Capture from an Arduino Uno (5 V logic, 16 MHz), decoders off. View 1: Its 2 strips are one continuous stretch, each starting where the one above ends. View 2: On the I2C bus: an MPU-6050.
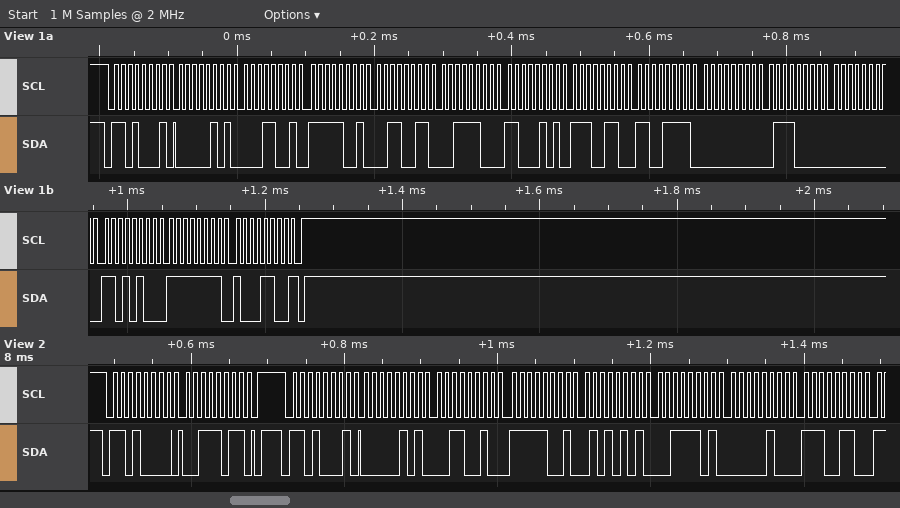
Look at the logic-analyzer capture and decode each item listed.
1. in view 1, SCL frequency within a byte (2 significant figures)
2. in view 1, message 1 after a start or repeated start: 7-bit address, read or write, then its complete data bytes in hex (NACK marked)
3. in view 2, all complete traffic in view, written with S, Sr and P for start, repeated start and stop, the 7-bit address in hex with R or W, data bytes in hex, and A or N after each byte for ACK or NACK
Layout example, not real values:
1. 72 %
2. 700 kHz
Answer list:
1. 100 kHz
2. 0x68 read: 05 19 F9 33 3C C5 E6 CF 00 70 00 D4 FF 8C NACK
3. S 68W A 3B A P S 68R A 05 A 32 A F9 A 55 A 3D A 04 A E6 A
